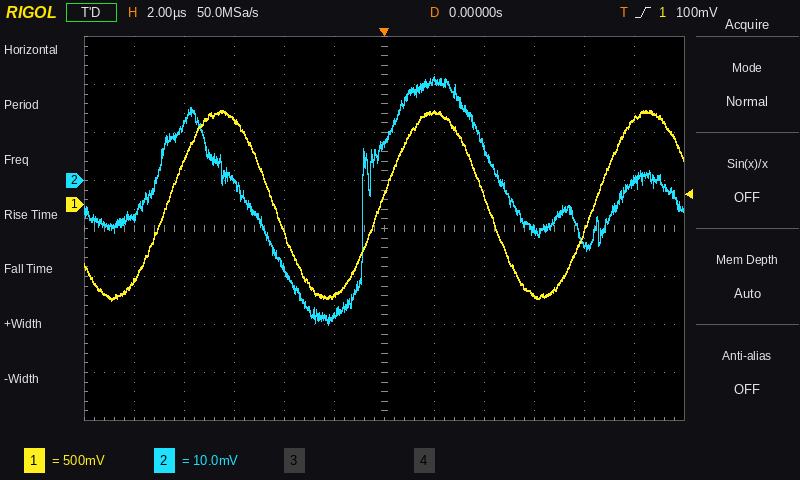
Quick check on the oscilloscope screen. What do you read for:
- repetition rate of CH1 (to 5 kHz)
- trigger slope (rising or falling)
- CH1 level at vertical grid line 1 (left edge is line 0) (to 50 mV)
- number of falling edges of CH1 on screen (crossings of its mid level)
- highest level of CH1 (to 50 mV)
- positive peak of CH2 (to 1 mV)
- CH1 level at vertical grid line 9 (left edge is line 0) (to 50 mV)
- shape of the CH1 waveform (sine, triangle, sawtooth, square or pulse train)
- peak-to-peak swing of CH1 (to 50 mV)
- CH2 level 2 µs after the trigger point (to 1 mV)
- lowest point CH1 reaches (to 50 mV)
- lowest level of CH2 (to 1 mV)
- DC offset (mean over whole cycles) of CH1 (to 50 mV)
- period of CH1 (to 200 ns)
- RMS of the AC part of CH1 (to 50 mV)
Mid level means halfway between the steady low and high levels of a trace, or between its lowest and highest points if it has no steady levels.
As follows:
115 kHz
rising
-800 mV
2
1.00 V
22 mV
-950 mV
sine
2.00 V
21 mV
-1.00 V
-30 mV
0 mV
8.6 µs
700 mV
